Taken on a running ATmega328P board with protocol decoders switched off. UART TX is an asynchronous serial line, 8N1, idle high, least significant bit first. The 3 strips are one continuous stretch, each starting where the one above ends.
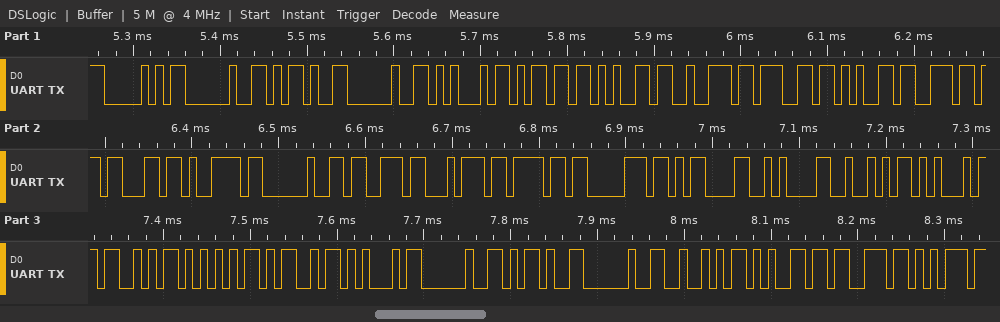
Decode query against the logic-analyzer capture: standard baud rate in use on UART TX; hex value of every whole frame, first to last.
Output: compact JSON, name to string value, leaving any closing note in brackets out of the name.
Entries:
{"standard baud rate in use on UART TX": "115200 baud", "hex value of every whole frame, first to last": "50 20 2D 20 45 6D 65 72 67 65 6E 63 79 20 73 74 6F 70 0D 0A 52 45 53 55 4D 45 20 2D 20 52 65 73 75"}
